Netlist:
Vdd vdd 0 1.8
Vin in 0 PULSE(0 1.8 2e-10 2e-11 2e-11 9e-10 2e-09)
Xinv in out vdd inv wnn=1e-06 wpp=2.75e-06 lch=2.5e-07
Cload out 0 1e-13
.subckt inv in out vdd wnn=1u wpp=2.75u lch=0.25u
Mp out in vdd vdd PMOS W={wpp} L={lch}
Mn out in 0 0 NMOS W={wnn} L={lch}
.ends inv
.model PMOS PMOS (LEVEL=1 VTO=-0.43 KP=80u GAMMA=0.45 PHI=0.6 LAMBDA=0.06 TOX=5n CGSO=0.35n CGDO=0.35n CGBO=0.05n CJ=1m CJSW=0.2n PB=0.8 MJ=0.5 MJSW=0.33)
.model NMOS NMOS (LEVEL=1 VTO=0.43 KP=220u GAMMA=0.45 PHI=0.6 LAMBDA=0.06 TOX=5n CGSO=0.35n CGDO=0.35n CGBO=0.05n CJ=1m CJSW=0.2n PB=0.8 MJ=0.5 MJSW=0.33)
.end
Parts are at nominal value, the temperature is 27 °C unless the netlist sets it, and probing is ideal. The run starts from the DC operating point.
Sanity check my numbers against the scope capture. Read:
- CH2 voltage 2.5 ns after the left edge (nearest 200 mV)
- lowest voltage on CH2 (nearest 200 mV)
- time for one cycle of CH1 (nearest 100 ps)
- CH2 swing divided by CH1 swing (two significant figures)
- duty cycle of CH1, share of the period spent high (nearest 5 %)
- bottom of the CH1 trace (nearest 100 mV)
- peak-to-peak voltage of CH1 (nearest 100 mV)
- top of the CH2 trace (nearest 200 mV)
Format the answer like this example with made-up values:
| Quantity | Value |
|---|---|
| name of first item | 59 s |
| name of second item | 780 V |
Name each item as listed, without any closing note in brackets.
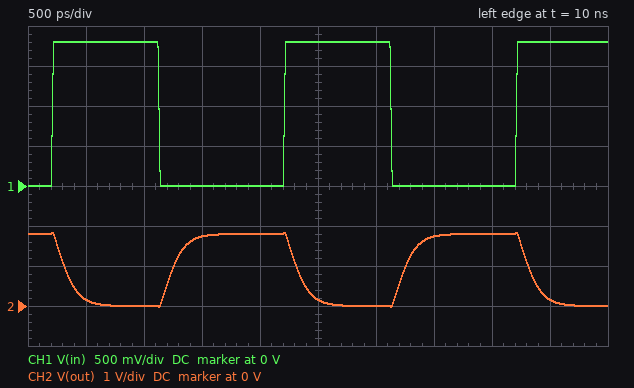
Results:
| Quantity | Value |
|---|---|
| CH2 voltage 2.5 ns after the left edge | 200 mV |
| lowest voltage on CH2 | 0 V |
| time for one cycle of CH1 | 2.0 ns |
| CH2 swing divided by CH1 swing | 1.0 |
| duty cycle of CH1, share of the period spent high | 45 % |
| bottom of the CH1 trace | 0 V |
| peak-to-peak voltage of CH1 | 1.8 V |
| top of the CH2 trace | 1.8 V |
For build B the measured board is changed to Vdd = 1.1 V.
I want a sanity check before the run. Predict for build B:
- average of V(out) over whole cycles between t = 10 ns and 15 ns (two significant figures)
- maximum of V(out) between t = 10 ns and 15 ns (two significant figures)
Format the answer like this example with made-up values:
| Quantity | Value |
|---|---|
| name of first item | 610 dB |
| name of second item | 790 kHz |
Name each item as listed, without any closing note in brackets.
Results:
| Quantity | Value |
|---|---|
| average of V(out) over whole cycles between t = 10 ns and 15 ns | 470 mV |
| maximum of V(out) between t = 10 ns and 15 ns | 1.1 V |
